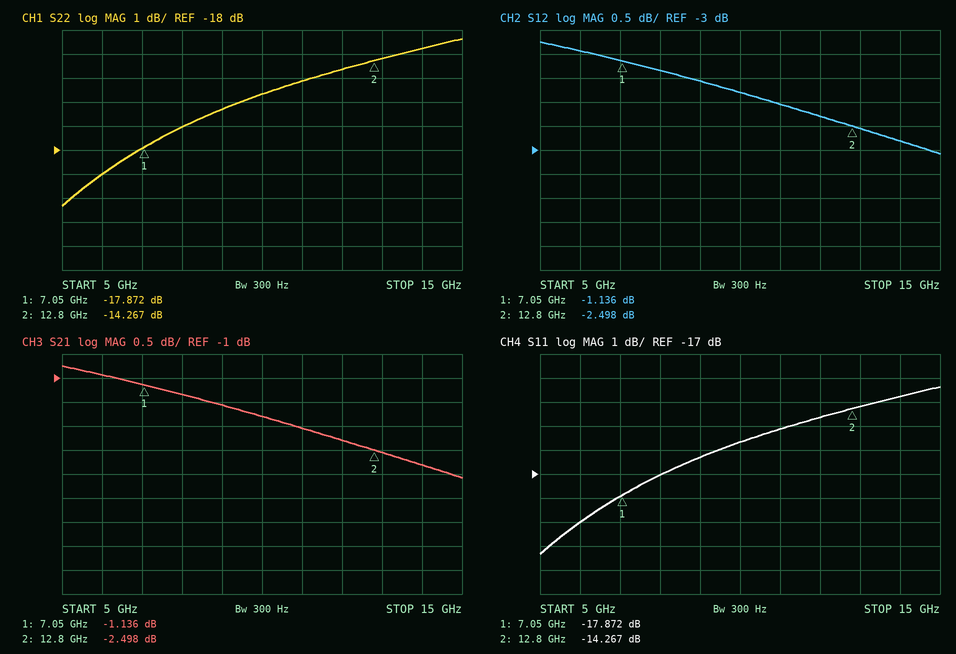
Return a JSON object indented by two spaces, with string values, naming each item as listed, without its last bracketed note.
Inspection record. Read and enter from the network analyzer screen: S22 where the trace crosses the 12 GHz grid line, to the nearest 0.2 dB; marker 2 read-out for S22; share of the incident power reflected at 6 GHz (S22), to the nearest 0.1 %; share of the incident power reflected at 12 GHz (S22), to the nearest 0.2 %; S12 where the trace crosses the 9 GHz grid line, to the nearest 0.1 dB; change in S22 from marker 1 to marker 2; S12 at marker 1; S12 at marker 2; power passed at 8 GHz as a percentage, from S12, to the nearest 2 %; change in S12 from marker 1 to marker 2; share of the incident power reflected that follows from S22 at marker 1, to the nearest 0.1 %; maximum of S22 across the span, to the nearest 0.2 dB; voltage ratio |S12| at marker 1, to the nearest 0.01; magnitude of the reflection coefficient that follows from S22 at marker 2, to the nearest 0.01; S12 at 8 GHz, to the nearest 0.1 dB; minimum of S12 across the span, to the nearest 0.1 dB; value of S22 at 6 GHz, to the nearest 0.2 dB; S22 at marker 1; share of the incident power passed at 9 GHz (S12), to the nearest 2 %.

{
  "S22 where the trace crosses the 12 GHz grid line, to the nearest 0.2 dB": "-14.6 dB",
  "marker 2 read-out for S22": "-14.267 dB",
  "share of the incident power reflected at 6 GHz (S22), to the nearest 0.1 %": "1.3 %",
  "share of the incident power reflected at 12 GHz (S22), to the nearest 0.2 %": "3.4 %",
  "S12 where the trace crosses the 9 GHz grid line, to the nearest 0.1 dB": "-1.6 dB",
  "change in S22 from marker 1 to marker 2": "3.605 dB",
  "S12 at marker 1": "-1.136 dB",
  "S12 at marker 2": "-2.498 dB",
  "power passed at 8 GHz as a percentage, from S12, to the nearest 2 %": "74 %",
  "change in S12 from marker 1 to marker 2": "-1.362 dB",
  "share of the incident power reflected that follows from S22 at marker 1, to the nearest 0.1 %": "1.6 %",
  "maximum of S22 across the span, to the nearest 0.2 dB": "-13.4 dB",
  "voltage ratio |S12| at marker 1, to the nearest 0.01": "0.88",
  "magnitude of the reflection coefficient that follows from S22 at marker 2, to the nearest 0.01": "0.19",
  "S12 at 8 GHz, to the nearest 0.1 dB": "-1.3 dB",
  "minimum of S12 across the span, to the nearest 0.1 dB": "-3.1 dB",
  "value of S22 at 6 GHz, to the nearest 0.2 dB": "-19.0 dB",
  "S22 at marker 1": "-17.872 dB",
  "share of the incident power passed at 9 GHz (S12), to the nearest 2 %": "70 %"
}
